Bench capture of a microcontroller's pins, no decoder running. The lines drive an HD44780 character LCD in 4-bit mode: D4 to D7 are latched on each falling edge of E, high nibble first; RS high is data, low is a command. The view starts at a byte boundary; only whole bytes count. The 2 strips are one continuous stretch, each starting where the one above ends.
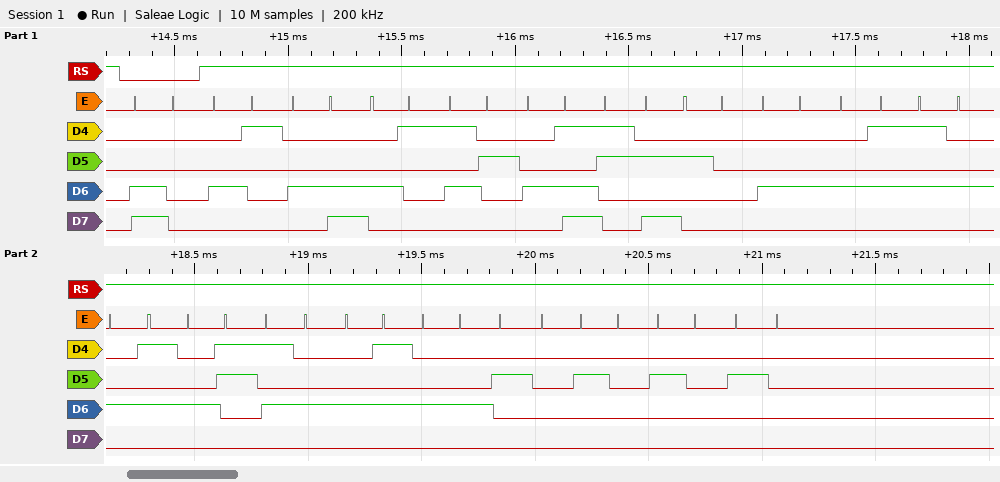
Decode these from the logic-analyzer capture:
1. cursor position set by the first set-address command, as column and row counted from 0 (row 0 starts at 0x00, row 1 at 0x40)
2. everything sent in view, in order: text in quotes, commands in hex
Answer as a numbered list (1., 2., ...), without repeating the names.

1. column 0, row 1
2. 0xC0 "ALARM: DETECTED    "
